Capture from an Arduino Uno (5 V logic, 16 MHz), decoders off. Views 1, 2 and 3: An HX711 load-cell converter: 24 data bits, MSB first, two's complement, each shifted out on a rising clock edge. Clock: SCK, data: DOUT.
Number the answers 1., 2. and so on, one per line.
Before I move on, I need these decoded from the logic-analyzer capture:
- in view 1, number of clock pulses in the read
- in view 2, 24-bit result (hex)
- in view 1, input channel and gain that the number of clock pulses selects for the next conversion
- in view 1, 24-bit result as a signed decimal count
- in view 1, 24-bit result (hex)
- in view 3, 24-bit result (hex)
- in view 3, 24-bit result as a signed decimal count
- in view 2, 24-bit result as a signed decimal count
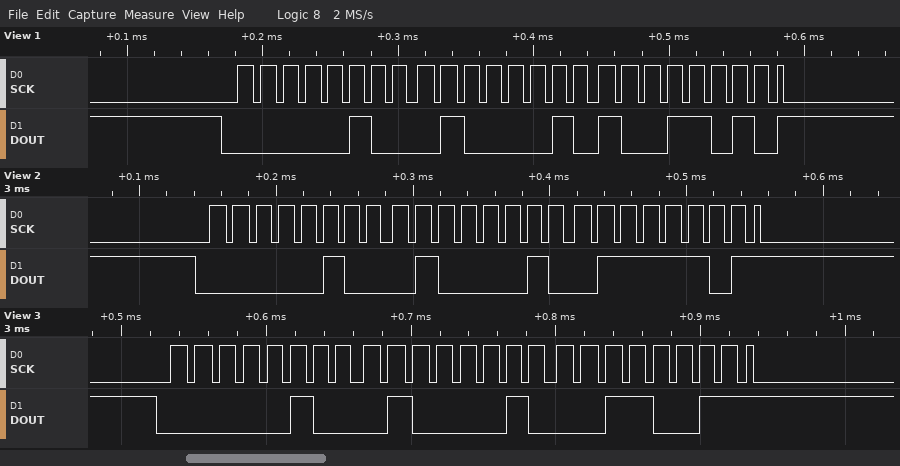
1. 25
2. 0x04427D
3. channel A, gain 128
4. 279194
5. 0x04429A
6. 0x044233
7. 279091
8. 279165
